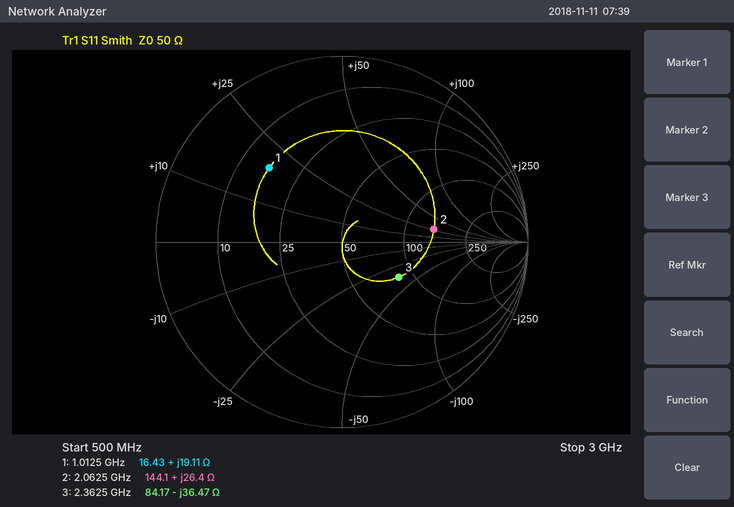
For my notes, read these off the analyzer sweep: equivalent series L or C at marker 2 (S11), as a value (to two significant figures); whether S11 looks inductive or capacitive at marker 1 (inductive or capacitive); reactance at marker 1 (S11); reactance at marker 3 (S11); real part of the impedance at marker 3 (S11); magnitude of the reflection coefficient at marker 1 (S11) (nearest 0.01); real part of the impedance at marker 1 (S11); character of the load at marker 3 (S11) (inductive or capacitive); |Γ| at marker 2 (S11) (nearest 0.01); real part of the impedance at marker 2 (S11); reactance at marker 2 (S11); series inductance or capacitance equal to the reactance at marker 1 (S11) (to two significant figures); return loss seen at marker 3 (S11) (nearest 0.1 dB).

2.0 nH
inductive
+19.11 Ω
-36.47 Ω
84.17 Ω
0.56
16.43 Ω
capacitive
0.50
144.1 Ω
+26.4 Ω
3.0 nH
8.9 dB
